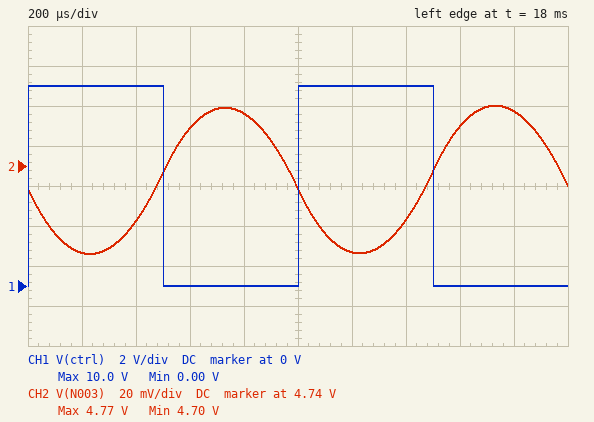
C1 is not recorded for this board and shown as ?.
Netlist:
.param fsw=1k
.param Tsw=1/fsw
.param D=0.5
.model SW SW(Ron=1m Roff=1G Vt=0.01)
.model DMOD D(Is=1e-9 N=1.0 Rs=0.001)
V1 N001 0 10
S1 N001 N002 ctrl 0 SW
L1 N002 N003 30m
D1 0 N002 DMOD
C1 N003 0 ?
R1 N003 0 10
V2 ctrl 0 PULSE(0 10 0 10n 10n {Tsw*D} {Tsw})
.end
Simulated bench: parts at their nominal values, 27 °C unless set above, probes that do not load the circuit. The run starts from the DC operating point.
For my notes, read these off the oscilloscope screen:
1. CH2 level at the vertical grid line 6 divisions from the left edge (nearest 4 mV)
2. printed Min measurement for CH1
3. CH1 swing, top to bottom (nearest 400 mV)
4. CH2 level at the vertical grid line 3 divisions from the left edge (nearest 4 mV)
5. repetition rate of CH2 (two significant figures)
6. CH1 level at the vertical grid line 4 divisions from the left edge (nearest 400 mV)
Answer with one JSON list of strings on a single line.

["4.696 V", "0.00 V", "10.0 V", "4.760 V", "1.0 kHz", "0 V"]
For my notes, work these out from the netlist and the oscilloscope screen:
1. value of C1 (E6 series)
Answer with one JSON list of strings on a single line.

["150 µF"]
